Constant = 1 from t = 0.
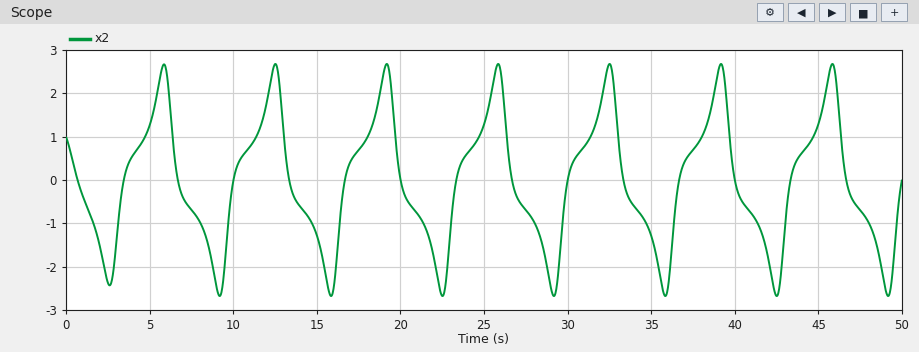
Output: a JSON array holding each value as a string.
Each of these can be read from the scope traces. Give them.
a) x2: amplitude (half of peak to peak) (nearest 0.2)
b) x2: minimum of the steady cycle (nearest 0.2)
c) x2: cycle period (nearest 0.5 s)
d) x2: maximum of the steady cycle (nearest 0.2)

["2.6", "-2.6", "6.5 s", "2.6"]
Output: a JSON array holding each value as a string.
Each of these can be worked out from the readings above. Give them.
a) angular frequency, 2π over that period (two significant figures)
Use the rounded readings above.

["0.97 rad/s"]
